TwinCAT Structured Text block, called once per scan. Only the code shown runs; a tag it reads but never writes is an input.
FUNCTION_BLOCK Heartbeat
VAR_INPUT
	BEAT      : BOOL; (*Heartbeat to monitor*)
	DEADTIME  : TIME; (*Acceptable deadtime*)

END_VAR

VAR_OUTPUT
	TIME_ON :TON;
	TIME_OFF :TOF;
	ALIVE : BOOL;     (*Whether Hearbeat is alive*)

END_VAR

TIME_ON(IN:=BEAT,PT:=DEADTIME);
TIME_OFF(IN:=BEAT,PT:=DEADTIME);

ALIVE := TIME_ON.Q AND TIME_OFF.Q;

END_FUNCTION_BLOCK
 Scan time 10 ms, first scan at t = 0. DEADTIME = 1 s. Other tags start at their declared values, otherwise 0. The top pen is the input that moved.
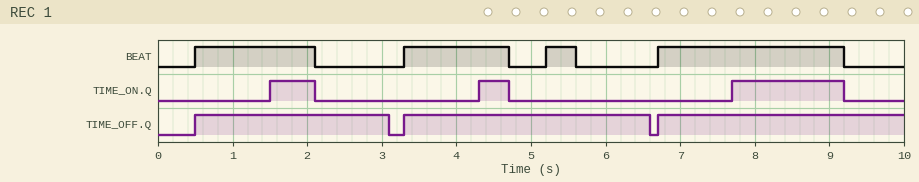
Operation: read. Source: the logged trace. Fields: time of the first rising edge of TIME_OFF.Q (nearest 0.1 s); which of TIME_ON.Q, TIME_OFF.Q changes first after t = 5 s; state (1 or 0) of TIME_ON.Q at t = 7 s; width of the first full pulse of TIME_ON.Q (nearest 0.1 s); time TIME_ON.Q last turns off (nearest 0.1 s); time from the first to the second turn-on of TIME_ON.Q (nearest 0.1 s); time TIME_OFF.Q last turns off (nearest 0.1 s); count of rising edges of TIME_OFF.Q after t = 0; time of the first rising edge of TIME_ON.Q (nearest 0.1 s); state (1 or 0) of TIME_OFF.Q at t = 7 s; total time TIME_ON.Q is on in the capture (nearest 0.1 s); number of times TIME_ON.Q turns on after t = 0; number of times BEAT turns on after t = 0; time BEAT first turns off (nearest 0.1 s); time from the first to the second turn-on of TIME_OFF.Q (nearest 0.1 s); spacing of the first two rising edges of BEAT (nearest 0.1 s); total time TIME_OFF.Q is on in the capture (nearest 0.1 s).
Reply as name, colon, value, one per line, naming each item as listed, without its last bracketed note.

time of the first rising edge of TIME_OFF.Q: 0.5 s
which of TIME_ON.Q, TIME_OFF.Q changes first after t = 5 s: TIME_OFF.Q
state (1 or 0) of TIME_ON.Q at t = 7 s: 0
width of the first full pulse of TIME_ON.Q: 0.6 s
time TIME_ON.Q last turns off: 9.2 s
time from the first to the second turn-on of TIME_ON.Q: 2.8 s
time TIME_OFF.Q last turns off: 6.6 s
count of rising edges of TIME_OFF.Q after t = 0: 3
time of the first rising edge of TIME_ON.Q: 1.5 s
state (1 or 0) of TIME_OFF.Q at t = 7 s: 1
total time TIME_ON.Q is on in the capture: 2.5 s
number of times TIME_ON.Q turns on after t = 0: 3
number of times BEAT turns on after t = 0: 4
time BEAT first turns off: 2.1 s
time from the first to the second turn-on of TIME_OFF.Q: 2.8 s
spacing of the first two rising edges of BEAT: 2.8 s
total time TIME_OFF.Q is on in the capture: 9.2 s
